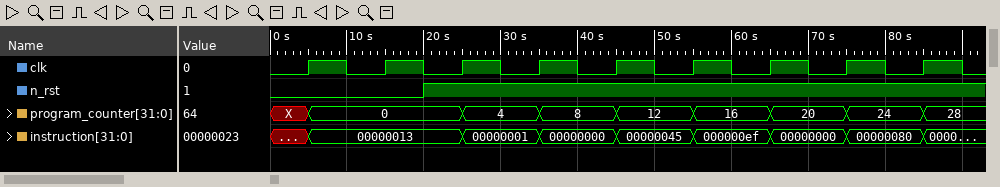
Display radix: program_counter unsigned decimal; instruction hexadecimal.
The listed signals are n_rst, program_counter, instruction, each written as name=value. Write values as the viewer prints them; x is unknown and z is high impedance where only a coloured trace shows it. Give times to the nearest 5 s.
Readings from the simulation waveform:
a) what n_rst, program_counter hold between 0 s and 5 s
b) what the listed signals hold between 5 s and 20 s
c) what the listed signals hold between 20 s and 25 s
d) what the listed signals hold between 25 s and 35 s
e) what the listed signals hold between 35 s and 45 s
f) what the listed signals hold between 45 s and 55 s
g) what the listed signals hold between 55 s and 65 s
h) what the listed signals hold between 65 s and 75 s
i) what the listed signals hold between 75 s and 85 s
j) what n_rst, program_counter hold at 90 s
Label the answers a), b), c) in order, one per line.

a) n_rst=0, program_counter=X
b) n_rst=0, program_counter=0, instruction=00000013
c) n_rst=1, program_counter=0, instruction=00000013
d) n_rst=1, program_counter=4, instruction=00000001
e) n_rst=1, program_counter=8, instruction=00000000
f) n_rst=1, program_counter=12, instruction=00000045
g) n_rst=1, program_counter=16, instruction=000000ef
h) n_rst=1, program_counter=20, instruction=00000000
i) n_rst=1, program_counter=24, instruction=00000080
j) n_rst=1, program_counter=28
